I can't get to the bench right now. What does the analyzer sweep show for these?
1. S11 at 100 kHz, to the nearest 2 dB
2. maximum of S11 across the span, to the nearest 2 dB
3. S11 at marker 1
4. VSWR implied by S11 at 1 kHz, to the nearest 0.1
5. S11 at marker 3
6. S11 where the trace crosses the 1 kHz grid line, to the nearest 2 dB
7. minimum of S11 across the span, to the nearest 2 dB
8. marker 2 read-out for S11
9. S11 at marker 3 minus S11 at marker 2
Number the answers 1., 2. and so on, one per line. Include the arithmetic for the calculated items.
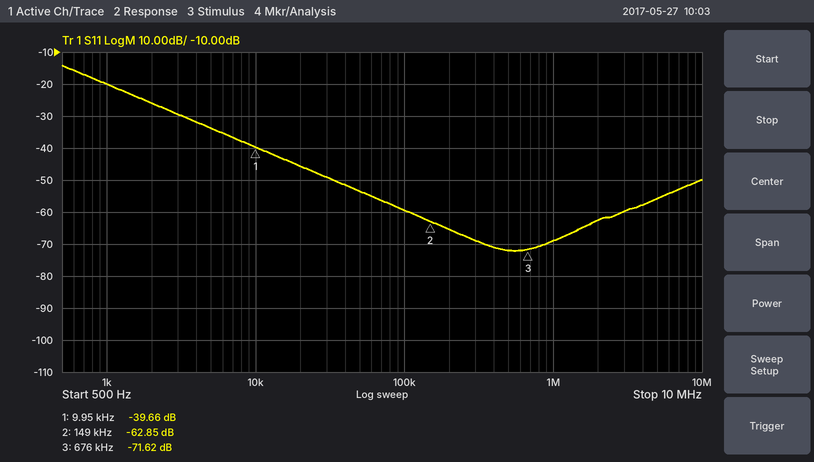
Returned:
1. -60 dB
2. -14 dB
3. -39.66 dB
4. |Γ| = 10^(-20/20) = 0.1000; VSWR = (1 + 0.1000)/(1 − 0.1000) ≈ 1.2
5. -71.62 dB
6. -20 dB
7. -72 dB
8. -62.85 dB
9. -71.62 − (-62.85) = -8.77 dB
